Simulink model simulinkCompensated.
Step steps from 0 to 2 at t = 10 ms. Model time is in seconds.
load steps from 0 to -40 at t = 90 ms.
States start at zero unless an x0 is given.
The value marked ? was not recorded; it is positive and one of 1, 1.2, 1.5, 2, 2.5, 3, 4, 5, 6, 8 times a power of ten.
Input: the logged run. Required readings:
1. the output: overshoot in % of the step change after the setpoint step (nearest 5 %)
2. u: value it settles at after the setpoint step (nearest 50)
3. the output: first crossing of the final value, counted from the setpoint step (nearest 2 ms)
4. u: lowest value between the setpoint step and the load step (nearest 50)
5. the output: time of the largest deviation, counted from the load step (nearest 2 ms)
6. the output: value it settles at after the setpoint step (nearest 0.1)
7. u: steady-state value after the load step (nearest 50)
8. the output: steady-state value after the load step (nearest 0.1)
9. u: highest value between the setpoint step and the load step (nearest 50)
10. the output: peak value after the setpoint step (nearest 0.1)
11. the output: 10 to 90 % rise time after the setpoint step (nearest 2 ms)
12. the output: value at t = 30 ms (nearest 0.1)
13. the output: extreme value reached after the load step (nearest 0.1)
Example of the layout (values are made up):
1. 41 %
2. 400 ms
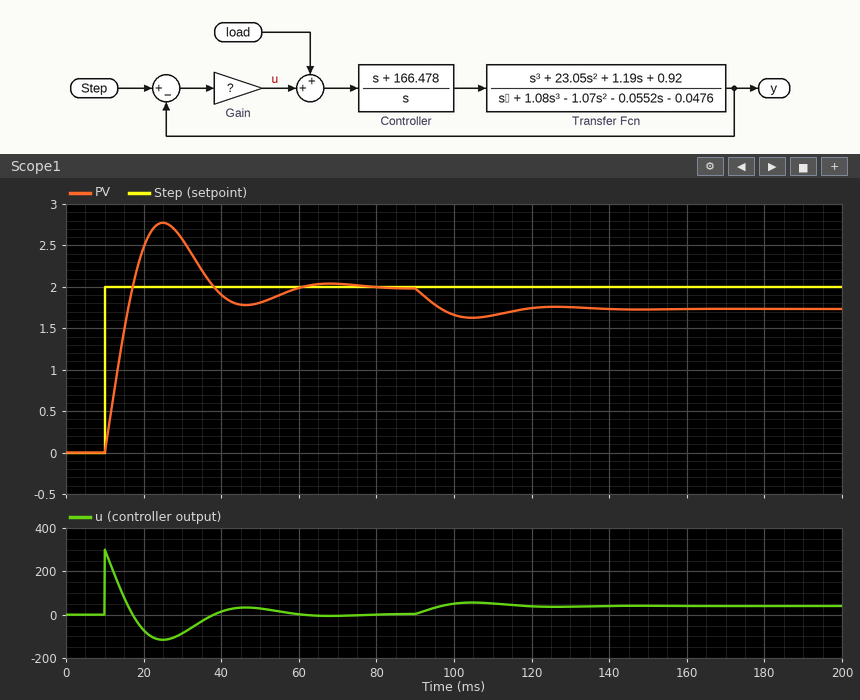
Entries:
1. 40 %
2. 0
3. 8 ms
4. -100
5. 14 ms
6. 2.0
7. 50
8. 1.7
9. 300
10. 2.8
11. 6 ms
12. 2.6
13. 1.6
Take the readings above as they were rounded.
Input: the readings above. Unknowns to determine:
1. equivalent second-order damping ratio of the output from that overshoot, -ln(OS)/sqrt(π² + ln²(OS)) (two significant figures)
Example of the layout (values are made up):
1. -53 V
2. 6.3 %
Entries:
1. 0.28
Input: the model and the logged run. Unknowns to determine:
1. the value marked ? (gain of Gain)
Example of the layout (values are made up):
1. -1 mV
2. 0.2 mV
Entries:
1. 150
